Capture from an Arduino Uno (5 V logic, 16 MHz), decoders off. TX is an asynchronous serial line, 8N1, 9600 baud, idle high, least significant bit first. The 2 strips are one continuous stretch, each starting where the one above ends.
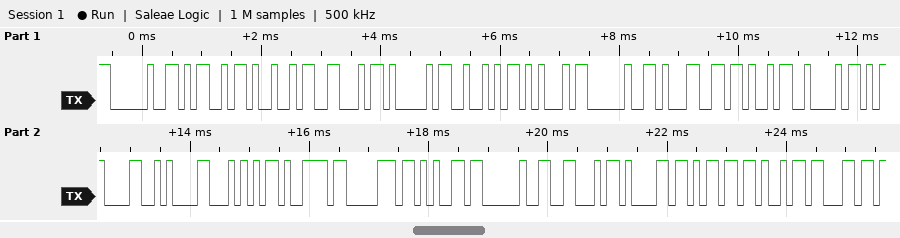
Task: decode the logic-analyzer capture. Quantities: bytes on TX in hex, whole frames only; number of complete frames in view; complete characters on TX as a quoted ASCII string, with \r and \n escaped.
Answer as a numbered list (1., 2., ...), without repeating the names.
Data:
1. 20 4D 49 46 41 52 45 20 31 4B 42 0D 0A 54 79 70 65 20 46 61 6D 69 6C
2. 23
3. " MIFARE 1KB\r\nType Famil"
